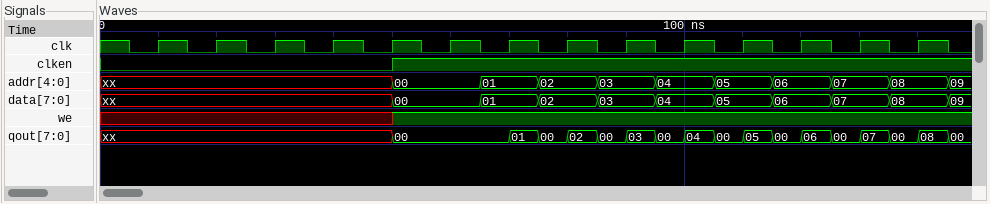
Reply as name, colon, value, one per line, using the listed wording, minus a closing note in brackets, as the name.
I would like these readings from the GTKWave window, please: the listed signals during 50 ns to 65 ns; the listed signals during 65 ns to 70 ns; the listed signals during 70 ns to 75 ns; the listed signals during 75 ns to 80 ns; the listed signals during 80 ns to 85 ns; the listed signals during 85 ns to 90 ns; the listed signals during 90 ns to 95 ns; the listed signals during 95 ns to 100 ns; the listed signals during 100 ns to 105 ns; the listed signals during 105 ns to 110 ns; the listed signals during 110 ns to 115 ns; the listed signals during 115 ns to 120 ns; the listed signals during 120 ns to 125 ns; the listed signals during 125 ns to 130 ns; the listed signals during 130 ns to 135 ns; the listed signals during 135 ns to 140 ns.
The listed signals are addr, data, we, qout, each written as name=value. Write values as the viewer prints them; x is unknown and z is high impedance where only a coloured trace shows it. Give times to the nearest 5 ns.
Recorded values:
the listed signals during 50 ns to 65 ns: addr=00, data=00, we=1, qout=00
the listed signals during 65 ns to 70 ns: addr=01, data=01, we=1, qout=00
the listed signals during 70 ns to 75 ns: addr=01, data=01, we=1, qout=01
the listed signals during 75 ns to 80 ns: addr=02, data=02, we=1, qout=00
the listed signals during 80 ns to 85 ns: addr=02, data=02, we=1, qout=02
the listed signals during 85 ns to 90 ns: addr=03, data=03, we=1, qout=00
the listed signals during 90 ns to 95 ns: addr=03, data=03, we=1, qout=03
the listed signals during 95 ns to 100 ns: addr=04, data=04, we=1, qout=00
the listed signals during 100 ns to 105 ns: addr=04, data=04, we=1, qout=04
the listed signals during 105 ns to 110 ns: addr=05, data=05, we=1, qout=00
the listed signals during 110 ns to 115 ns: addr=05, data=05, we=1, qout=05
the listed signals during 115 ns to 120 ns: addr=06, data=06, we=1, qout=00
the listed signals during 120 ns to 125 ns: addr=06, data=06, we=1, qout=06
the listed signals during 125 ns to 130 ns: addr=07, data=07, we=1, qout=00
the listed signals during 130 ns to 135 ns: addr=07, data=07, we=1, qout=07
the listed signals during 135 ns to 140 ns: addr=08, data=08, we=1, qout=00
